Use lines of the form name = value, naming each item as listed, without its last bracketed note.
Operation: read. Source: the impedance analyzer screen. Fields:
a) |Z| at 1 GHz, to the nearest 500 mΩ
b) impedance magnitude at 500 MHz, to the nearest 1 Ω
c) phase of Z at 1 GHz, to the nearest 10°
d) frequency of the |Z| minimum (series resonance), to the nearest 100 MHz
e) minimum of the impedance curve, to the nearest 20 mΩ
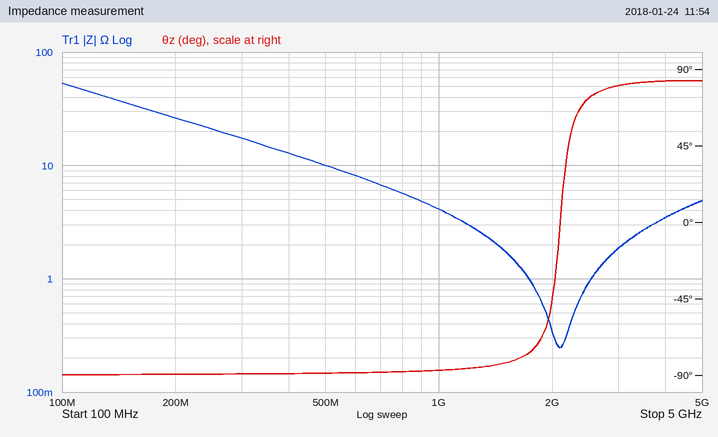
|Z| at 1 GHz, to the nearest 500 mΩ = 4.0 Ω
impedance magnitude at 500 MHz, to the nearest 1 Ω = 10 Ω
phase of Z at 1 GHz, to the nearest 10° = -90°
frequency of the |Z| minimum (series resonance), to the nearest 100 MHz = 2.1 GHz
minimum of the impedance curve, to the nearest 20 mΩ = 240 mΩ
